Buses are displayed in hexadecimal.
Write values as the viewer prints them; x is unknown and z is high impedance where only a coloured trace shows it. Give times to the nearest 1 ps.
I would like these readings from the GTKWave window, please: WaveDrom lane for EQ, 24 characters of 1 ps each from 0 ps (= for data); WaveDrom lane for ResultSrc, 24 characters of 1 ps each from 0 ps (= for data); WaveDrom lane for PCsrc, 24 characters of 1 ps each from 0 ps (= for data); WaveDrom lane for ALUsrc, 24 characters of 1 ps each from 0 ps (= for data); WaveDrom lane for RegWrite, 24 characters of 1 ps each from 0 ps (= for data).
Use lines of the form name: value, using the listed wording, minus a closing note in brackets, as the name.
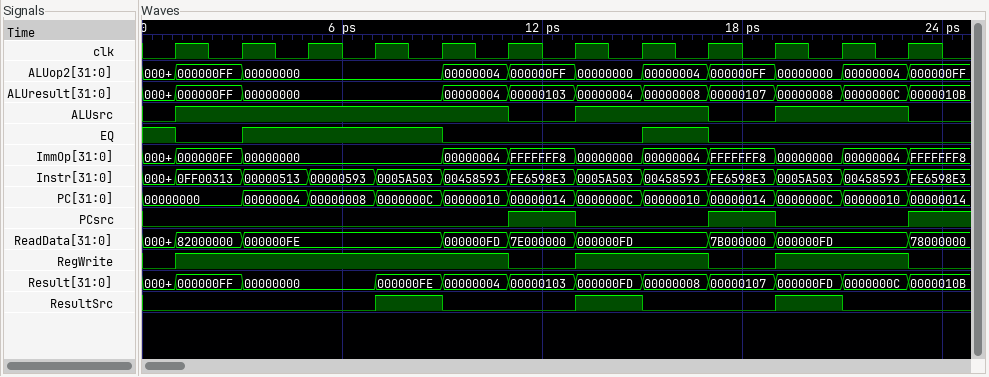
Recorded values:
WaveDrom lane for EQ, 24 characters of 1 ps each from 0 ps: {name: 'EQ', wave: '10.1.....0.....1.0......'}
WaveDrom lane for ResultSrc, 24 characters of 1 ps each from 0 ps: {name: 'ResultSrc', wave: '0......1.0...1.0...1.0..'}
WaveDrom lane for PCsrc, 24 characters of 1 ps each from 0 ps: {name: 'PCsrc', wave: '0..........1.0...1.0...1'}
WaveDrom lane for ALUsrc, 24 characters of 1 ps each from 0 ps: {name: 'ALUsrc', wave: '01.........0.1...0.1...0'}
WaveDrom lane for RegWrite, 24 characters of 1 ps each from 0 ps: {name: 'RegWrite', wave: '01.........0.1...0.1...0'}
